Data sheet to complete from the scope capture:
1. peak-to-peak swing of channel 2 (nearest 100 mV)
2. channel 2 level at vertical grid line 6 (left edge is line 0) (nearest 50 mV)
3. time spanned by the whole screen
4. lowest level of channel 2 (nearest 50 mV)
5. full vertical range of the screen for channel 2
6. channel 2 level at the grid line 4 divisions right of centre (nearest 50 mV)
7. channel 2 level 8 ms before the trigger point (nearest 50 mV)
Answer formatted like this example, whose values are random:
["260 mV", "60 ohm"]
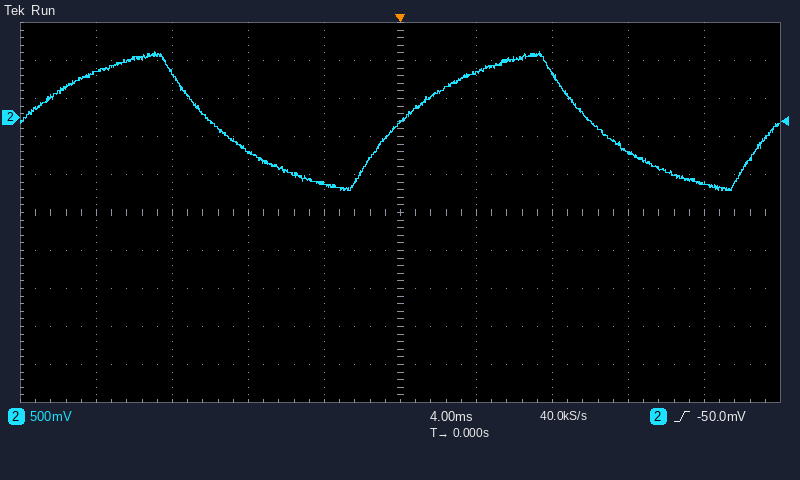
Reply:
["1.80 V", "600 mV", "40 ms", "-950 mV", "5 V", "-850 mV", "-450 mV"]
